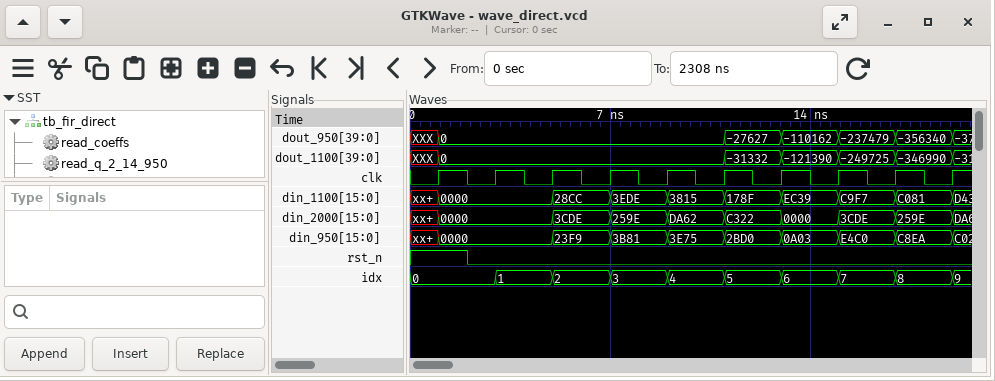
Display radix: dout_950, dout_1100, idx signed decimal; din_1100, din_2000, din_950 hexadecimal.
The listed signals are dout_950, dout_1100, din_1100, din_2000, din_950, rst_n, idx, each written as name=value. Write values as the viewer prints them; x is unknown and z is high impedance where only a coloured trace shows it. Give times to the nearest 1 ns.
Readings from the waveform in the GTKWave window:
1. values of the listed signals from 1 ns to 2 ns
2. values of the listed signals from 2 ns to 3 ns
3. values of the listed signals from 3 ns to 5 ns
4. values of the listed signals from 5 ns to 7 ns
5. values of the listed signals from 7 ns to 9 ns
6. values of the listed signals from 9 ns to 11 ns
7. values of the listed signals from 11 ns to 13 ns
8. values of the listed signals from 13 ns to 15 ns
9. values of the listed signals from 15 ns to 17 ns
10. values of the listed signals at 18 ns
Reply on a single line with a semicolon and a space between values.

dout_950=0, dout_1100=0, din_1100=0000, din_2000=0000, din_950=0000, rst_n=1, idx=0; dout_950=0, dout_1100=0, din_1100=0000, din_2000=0000, din_950=0000, rst_n=0, idx=0; dout_950=0, dout_1100=0, din_1100=0000, din_2000=0000, din_950=0000, rst_n=0, idx=1; dout_950=0, dout_1100=0, din_1100=28CC, din_2000=3CDE, din_950=23F9, rst_n=0, idx=2; dout_950=0, dout_1100=0, din_1100=3EDE, din_2000=259E, din_950=3B81, rst_n=0, idx=3; dout_950=0, dout_1100=0, din_1100=3815, din_2000=DA62, din_950=3E75, rst_n=0, idx=4; dout_950=-27627, dout_1100=-31332, din_1100=178F, din_2000=C322, din_950=2BD0, rst_n=0, idx=5; dout_950=-110162, dout_1100=-121390, din_1100=EC39, din_2000=0000, din_950=0A03, rst_n=0, idx=6; dout_950=-237479, dout_1100=-249725, din_1100=C9F7, din_2000=3CDE, din_950=E4C0, rst_n=0, idx=7; dout_950=-356340, dout_1100=-346990, din_1100=C081, din_2000=259E, din_950=C8EA, rst_n=0, idx=8
